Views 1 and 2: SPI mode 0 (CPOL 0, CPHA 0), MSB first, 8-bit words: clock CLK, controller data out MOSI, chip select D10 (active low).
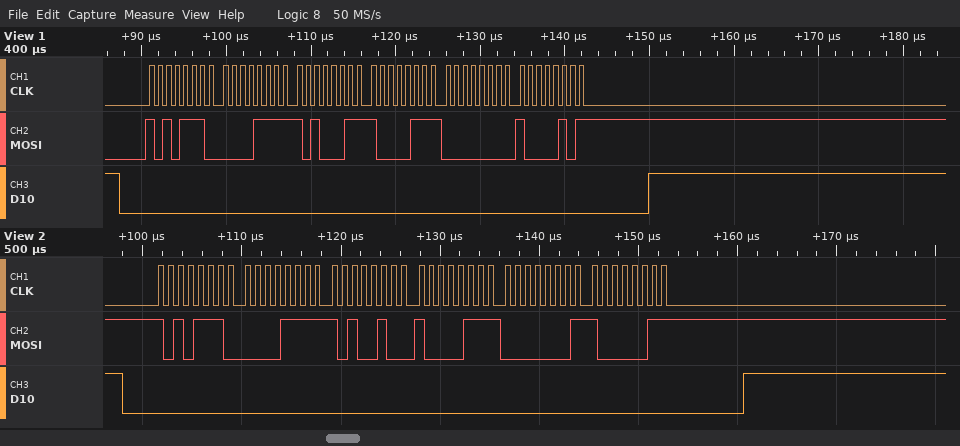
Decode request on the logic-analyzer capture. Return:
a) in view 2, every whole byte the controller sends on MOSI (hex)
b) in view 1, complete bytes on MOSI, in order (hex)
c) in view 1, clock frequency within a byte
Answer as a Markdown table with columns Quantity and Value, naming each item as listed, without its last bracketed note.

| Quantity | Value |
|---|---|
| in view 2, every whole byte the controller sends on MOSI | AE 0F A4 87 01 83 |
| in view 1, complete bytes on MOSI, in order | AE 0F A3 87 00 85 |
| in view 1, clock frequency within a byte | 1 MHz |
